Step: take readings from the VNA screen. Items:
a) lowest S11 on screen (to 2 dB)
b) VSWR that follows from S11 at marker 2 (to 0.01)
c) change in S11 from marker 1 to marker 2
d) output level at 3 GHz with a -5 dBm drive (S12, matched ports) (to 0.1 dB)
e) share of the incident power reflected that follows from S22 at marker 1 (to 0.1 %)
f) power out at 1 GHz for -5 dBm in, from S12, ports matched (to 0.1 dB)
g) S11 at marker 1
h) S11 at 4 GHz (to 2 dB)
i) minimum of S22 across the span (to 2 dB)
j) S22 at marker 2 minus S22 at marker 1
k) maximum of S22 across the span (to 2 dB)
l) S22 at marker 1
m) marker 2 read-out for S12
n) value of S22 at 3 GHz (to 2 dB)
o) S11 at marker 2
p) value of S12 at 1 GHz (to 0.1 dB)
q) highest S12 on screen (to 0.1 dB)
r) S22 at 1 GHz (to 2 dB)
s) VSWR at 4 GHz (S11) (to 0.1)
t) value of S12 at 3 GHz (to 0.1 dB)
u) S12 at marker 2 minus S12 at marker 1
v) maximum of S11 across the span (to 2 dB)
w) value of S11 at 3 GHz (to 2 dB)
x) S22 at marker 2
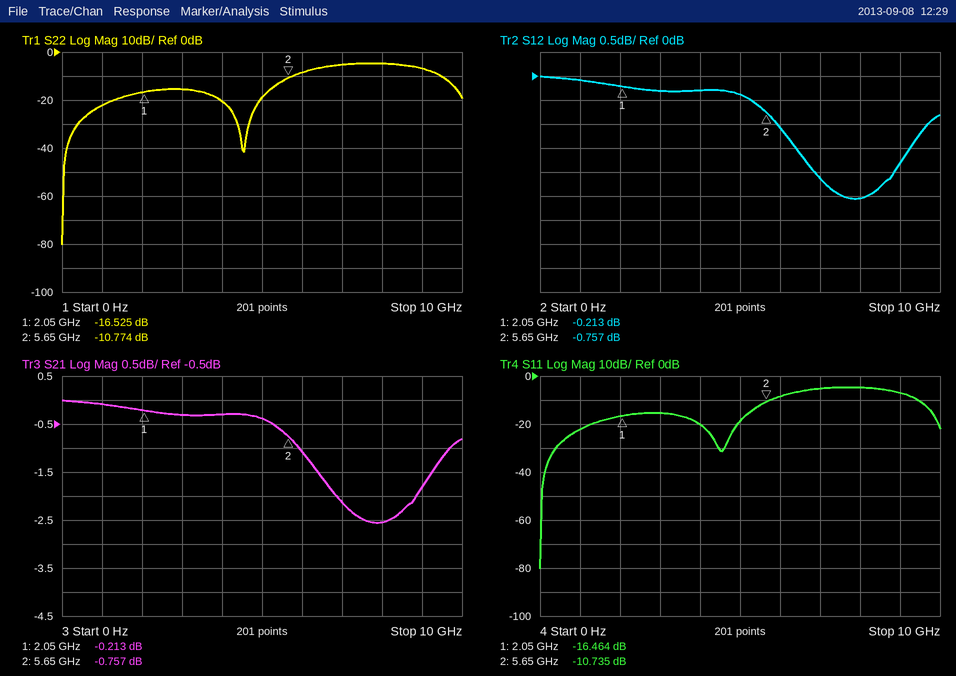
-80 dB
1.82
5.729 dB
-5.3 dBm
2.2 %
-5.1 dBm
-16.464 dB
-20 dB
-80 dB
5.751 dB
-4 dB
-16.525 dB
-0.757 dB
-16 dB
-10.735 dB
-0.1 dB
0.0 dB
-22 dB
1.2
-0.3 dB
-0.544 dB
-4 dB
-16 dB
-10.774 dB
